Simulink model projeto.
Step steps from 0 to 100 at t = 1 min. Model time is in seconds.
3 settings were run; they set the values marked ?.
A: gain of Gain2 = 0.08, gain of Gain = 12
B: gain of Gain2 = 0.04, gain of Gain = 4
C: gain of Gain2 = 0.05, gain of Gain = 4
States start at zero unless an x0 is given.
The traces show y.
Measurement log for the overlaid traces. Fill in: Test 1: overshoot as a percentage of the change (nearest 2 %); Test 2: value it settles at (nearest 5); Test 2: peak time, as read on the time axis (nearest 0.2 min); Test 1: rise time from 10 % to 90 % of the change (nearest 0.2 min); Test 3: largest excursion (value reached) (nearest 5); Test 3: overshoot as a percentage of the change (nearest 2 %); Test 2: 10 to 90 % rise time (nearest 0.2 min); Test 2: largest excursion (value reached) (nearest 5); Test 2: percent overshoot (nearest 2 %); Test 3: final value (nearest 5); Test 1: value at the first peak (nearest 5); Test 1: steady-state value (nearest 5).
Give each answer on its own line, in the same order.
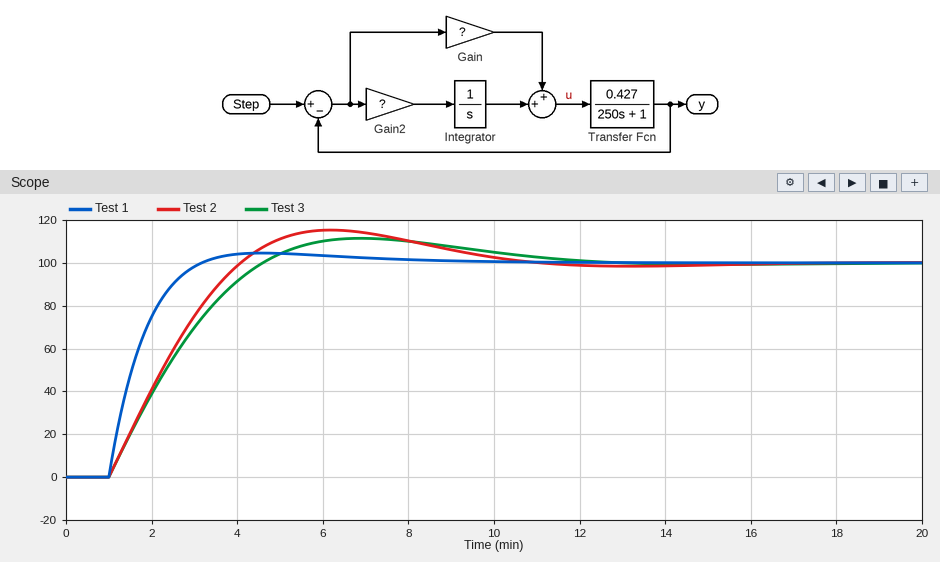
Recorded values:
4 %
100
6.2 min
1.4 min
110
12 %
2.4 min
115
16 %
100
105
100
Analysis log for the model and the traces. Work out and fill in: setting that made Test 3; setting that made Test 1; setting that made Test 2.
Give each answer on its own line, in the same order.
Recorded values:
B
A
C
